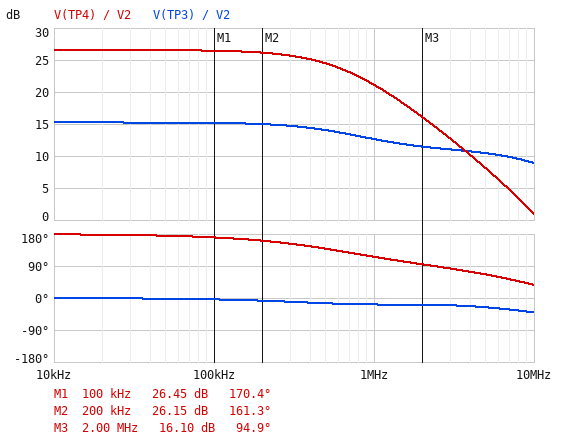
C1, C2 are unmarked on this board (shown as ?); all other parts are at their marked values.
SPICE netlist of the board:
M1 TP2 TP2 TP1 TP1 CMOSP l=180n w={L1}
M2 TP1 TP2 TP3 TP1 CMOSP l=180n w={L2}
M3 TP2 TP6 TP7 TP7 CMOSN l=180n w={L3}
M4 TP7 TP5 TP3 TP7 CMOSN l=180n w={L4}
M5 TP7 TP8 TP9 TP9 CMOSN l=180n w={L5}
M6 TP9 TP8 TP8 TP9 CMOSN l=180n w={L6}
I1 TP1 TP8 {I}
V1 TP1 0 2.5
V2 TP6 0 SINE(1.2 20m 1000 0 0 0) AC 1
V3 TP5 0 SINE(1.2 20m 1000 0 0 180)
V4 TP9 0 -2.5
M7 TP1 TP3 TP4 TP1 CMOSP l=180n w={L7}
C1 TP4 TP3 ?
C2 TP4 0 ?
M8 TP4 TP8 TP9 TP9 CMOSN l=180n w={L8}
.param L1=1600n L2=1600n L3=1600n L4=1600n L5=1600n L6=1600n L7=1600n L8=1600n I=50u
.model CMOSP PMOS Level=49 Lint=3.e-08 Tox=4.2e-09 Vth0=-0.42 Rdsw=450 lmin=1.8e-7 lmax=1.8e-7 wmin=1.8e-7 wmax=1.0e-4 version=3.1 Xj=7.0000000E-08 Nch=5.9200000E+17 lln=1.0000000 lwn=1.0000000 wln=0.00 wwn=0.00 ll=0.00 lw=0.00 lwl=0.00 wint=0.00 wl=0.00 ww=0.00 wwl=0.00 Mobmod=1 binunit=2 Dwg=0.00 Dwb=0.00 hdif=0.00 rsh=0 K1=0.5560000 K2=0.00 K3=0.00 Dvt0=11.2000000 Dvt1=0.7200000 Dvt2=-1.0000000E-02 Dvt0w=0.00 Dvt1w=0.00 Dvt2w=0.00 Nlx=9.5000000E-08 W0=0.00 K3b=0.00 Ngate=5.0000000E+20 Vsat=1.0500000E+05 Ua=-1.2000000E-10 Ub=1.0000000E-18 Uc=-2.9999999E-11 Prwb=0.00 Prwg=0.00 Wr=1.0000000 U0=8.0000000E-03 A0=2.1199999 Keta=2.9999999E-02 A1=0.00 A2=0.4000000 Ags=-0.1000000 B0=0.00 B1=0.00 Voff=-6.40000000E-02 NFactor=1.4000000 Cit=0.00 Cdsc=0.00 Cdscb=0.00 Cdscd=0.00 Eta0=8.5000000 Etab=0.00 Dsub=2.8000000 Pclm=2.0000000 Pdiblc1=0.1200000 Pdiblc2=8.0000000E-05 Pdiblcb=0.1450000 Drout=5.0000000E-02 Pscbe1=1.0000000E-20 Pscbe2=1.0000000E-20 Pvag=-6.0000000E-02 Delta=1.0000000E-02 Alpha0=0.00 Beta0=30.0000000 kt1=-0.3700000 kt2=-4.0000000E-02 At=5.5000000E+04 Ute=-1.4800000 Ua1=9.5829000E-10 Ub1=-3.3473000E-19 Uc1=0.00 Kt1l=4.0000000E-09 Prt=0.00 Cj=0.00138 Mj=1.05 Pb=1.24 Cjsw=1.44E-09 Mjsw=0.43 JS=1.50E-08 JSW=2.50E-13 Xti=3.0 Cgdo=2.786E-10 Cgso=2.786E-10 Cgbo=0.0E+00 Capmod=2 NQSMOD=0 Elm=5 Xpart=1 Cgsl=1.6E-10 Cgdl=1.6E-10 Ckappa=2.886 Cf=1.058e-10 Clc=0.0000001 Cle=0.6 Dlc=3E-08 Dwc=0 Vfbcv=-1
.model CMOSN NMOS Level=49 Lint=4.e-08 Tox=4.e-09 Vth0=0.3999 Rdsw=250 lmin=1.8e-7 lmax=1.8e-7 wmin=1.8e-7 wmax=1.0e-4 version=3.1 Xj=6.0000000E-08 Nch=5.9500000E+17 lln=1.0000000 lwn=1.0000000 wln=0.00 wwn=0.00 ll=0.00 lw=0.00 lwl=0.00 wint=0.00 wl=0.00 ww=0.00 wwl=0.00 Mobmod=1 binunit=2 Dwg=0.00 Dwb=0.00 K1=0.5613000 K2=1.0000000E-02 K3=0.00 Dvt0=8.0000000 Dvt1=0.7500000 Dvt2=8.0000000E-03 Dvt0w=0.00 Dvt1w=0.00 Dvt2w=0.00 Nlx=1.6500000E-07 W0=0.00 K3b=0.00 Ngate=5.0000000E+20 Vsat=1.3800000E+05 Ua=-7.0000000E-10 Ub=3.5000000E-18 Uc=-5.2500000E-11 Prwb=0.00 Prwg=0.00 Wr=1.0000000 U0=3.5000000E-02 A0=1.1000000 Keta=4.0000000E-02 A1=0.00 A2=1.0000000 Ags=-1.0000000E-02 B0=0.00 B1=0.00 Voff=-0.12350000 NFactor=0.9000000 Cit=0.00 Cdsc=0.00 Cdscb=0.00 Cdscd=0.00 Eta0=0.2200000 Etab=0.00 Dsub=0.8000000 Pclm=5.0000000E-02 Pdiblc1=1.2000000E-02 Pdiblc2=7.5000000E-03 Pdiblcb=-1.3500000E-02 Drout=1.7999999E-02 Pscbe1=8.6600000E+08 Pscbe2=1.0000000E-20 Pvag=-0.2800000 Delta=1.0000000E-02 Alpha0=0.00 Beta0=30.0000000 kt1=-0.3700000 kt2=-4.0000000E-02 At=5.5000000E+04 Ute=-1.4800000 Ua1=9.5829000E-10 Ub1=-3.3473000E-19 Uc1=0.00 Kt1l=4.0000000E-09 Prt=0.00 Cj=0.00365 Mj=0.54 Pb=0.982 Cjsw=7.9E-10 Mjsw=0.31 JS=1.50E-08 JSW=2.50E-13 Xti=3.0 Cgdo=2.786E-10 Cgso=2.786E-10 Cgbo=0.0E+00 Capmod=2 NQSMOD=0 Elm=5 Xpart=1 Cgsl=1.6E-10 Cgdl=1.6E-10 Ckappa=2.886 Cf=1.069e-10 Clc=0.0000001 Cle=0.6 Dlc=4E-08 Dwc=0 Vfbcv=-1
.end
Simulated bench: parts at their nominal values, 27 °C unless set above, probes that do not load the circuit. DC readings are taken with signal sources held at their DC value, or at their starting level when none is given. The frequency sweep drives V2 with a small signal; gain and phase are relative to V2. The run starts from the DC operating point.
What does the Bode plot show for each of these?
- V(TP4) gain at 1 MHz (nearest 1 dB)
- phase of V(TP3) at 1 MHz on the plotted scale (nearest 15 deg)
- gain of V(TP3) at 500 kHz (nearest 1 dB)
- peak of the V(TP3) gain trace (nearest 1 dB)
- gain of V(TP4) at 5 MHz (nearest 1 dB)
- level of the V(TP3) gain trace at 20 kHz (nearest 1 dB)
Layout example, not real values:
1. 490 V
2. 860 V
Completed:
1. 21 dB
2. -15 deg
3. 14 dB
4. 15 dB
5. 8 dB
6. 15 dB
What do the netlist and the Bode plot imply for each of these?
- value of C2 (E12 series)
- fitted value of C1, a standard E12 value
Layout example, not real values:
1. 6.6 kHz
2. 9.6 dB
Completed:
1. 15 pF
2. 2.2 pF
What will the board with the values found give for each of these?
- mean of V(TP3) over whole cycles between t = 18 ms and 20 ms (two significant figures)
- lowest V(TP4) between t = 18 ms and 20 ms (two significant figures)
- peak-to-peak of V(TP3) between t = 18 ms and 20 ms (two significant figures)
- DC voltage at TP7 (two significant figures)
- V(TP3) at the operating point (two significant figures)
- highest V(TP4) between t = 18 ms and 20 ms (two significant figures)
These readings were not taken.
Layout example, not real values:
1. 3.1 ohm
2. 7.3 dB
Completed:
1. 1.7 V
2. -870 mV
3. 460 mV
4. 600 mV
5. 1.7 V
6. 900 mV
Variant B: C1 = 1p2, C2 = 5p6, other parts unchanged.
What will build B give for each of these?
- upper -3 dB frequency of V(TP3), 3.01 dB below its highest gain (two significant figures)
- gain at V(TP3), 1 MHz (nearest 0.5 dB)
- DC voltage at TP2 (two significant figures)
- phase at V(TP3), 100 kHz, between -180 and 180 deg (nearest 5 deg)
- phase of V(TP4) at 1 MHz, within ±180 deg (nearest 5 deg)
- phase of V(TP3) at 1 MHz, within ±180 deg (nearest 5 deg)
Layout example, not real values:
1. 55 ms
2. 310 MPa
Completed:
1. 2.1 MHz
2. 14.0 dB
3. 1.7 V
4. 0 deg
5. 140 deg
6. -15 deg
